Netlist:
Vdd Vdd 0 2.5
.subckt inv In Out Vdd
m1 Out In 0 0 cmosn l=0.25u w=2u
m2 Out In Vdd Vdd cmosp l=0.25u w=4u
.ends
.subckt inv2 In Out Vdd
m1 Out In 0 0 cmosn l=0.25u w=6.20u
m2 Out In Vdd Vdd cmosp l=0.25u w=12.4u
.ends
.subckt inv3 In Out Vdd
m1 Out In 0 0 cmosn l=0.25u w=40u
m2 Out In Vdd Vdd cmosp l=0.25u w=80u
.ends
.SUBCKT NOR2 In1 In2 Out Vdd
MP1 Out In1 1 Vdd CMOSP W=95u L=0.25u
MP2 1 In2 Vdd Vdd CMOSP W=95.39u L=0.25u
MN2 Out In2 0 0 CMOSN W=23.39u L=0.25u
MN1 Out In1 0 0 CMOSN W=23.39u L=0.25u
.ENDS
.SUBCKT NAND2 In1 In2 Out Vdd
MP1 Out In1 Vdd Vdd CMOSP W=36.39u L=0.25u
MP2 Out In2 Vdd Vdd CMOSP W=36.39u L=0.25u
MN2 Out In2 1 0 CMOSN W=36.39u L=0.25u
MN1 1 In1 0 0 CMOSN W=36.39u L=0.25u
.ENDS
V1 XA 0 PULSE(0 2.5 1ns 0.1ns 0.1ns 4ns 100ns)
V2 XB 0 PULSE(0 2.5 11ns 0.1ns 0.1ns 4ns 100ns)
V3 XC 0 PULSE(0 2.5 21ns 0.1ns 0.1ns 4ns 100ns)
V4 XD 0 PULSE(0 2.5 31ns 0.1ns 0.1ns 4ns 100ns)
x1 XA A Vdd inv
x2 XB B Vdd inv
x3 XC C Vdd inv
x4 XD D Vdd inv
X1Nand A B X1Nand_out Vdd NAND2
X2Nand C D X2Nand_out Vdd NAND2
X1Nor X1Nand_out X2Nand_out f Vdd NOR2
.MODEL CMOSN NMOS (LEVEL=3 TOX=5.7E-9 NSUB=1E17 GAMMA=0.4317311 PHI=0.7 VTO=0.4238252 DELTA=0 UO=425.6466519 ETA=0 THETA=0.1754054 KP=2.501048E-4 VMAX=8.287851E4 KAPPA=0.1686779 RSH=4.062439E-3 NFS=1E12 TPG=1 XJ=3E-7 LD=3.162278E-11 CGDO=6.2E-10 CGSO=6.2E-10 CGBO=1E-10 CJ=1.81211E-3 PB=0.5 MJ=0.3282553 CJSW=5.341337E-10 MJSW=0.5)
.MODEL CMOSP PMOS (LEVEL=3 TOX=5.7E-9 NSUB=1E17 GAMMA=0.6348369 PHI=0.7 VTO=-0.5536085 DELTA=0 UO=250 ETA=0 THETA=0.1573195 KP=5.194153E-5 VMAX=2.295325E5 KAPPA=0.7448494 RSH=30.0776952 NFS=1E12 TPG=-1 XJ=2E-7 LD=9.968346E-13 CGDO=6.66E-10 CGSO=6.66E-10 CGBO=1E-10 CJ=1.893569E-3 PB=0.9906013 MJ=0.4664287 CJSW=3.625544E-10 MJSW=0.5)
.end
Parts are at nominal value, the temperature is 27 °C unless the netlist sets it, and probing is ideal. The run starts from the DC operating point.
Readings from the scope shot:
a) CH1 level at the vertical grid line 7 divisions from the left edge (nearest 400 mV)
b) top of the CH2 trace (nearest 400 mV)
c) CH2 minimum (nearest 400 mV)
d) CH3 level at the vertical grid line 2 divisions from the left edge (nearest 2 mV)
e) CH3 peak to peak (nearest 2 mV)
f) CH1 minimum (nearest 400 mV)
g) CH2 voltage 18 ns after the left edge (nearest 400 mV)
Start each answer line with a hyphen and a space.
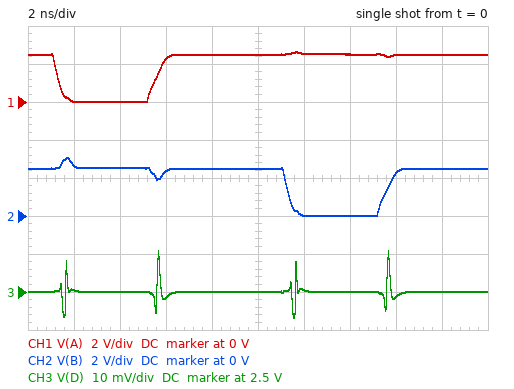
- 2.4 V
- 3.2 V
- 0 V
- 2.500 V
- 18 mV
- 0 V
- 2.4 V
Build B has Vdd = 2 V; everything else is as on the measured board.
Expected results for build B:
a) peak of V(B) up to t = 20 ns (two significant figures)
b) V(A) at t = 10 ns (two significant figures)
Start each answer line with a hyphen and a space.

- 2.5 V
- 2.0 V
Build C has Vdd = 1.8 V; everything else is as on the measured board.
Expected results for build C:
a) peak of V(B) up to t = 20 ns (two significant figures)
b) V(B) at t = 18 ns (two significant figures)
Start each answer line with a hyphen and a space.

- 2.2 V
- 1.8 V
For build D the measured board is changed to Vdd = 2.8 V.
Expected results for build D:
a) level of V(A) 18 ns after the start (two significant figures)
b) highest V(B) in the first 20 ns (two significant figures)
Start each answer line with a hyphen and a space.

- 2.8 V
- 3.4 V
